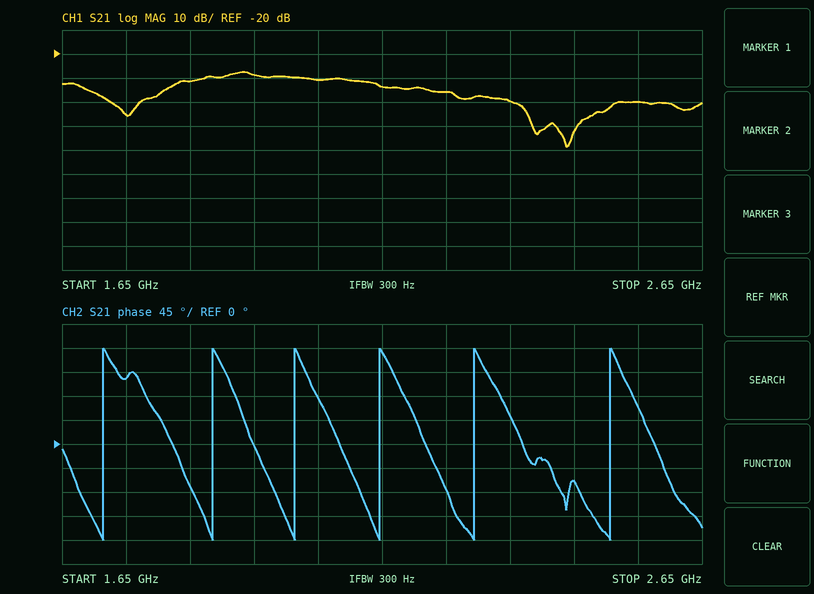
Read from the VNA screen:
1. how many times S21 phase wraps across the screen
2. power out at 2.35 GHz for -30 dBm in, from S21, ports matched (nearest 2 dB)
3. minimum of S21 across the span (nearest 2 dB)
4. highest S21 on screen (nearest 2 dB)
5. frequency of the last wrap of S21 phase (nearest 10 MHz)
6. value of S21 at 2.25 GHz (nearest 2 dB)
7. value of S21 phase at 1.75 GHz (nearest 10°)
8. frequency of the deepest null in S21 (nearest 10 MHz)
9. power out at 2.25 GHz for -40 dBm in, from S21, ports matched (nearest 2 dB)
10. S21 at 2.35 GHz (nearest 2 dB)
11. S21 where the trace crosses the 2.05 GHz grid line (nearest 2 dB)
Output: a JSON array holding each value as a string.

["6", "-70 dBm", "-58 dB", "-28 dB", "2.51 GHz", "-36 dB", "120°", "2.44 GHz", "-76 dBm", "-40 dB", "-30 dB"]
